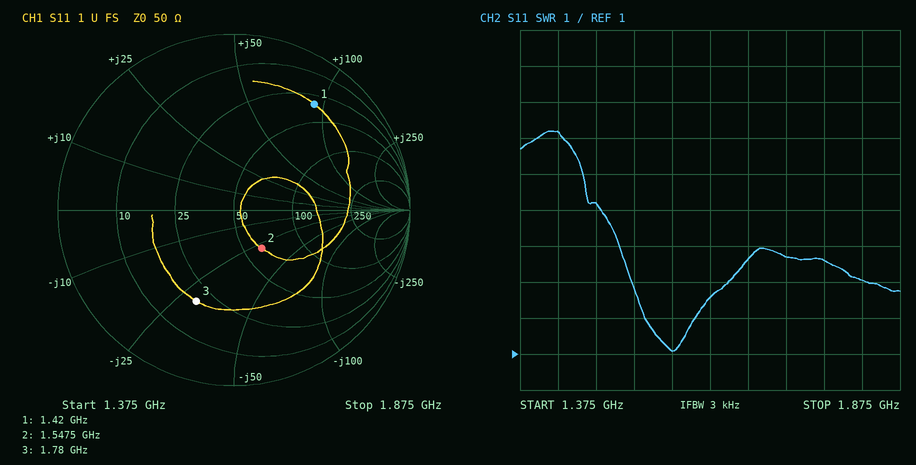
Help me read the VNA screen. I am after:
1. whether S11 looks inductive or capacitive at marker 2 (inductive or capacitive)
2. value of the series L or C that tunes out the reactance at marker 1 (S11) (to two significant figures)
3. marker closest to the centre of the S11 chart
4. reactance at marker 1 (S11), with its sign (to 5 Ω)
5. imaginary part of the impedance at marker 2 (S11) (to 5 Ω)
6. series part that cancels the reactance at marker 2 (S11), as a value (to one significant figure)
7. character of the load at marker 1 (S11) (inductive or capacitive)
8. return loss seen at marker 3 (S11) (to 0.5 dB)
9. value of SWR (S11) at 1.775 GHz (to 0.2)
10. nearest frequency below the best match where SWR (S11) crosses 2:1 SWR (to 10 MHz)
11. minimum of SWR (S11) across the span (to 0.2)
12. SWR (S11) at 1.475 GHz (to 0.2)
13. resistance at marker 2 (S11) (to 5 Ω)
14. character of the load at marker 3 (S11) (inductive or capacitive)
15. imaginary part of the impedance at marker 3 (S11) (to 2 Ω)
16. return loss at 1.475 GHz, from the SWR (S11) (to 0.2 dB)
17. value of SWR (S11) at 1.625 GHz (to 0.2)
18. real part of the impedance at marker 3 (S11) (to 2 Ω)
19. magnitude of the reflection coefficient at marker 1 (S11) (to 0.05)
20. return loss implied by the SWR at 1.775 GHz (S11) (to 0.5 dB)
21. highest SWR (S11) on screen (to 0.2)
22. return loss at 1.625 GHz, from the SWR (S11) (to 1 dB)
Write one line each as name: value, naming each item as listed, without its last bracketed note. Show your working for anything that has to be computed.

whether S11 looks inductive or capacitive at marker 2: capacitive
value of the series L or C that tunes out the reactance at marker 1 (S11): C = 1/(2π × 1.42 GHz × 90 Ω) ≈ 1.2 pF
marker closest to the centre of the S11 chart: marker 2
reactance at marker 1 (S11), with its sign: +90 Ω
imaginary part of the impedance at marker 2 (S11): -30 Ω
series part that cancels the reactance at marker 2 (S11), as a value: L = 30 Ω/(2π × 1.5475 GHz) ≈ 3 nH
character of the load at marker 1 (S11): inductive
return loss seen at marker 3 (S11): 5.0 dB
value of SWR (S11) at 1.775 GHz: 3.6
nearest frequency below the best match where SWR (S11) crosses 2:1 SWR: 1.54 GHz
minimum of SWR (S11) across the span: 1.0
SWR (S11) at 1.475 GHz: 5.2
resistance at marker 2 (S11): 60 Ω
character of the load at marker 3 (S11): capacitive
imaginary part of the impedance at marker 3 (S11): -30 Ω
return loss at 1.475 GHz, from the SWR (S11): −20 log10((5.2 − 1)/(5.2 + 1)) ≈ 3.4 dB
value of SWR (S11) at 1.625 GHz: 2.6
real part of the impedance at marker 3 (S11): 20 Ω
magnitude of the reflection coefficient at marker 1 (S11): 0.75
return loss implied by the SWR at 1.775 GHz (S11): −20 log10((3.6 − 1)/(3.6 + 1)) ≈ 5.0 dB
highest SWR (S11) on screen: 7.2
return loss at 1.625 GHz, from the SWR (S11): −20 log10((2.6 − 1)/(2.6 + 1)) ≈ 7 dB
